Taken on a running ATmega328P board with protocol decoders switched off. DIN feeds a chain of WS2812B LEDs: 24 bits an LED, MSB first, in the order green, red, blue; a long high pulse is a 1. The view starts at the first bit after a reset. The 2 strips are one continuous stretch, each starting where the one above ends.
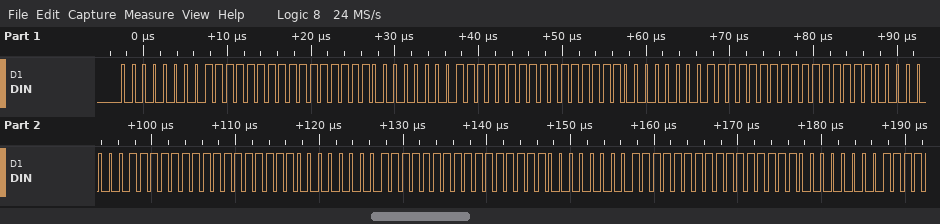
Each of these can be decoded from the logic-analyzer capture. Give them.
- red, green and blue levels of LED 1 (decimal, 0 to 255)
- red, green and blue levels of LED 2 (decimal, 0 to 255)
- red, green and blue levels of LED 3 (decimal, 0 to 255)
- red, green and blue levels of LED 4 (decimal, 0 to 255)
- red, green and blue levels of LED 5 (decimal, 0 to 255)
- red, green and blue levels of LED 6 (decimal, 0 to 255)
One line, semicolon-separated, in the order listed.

255, 0, 255; 255, 0, 255; 255, 0, 255; 255, 0, 255; 255, 0, 255; 255, 0, 255
